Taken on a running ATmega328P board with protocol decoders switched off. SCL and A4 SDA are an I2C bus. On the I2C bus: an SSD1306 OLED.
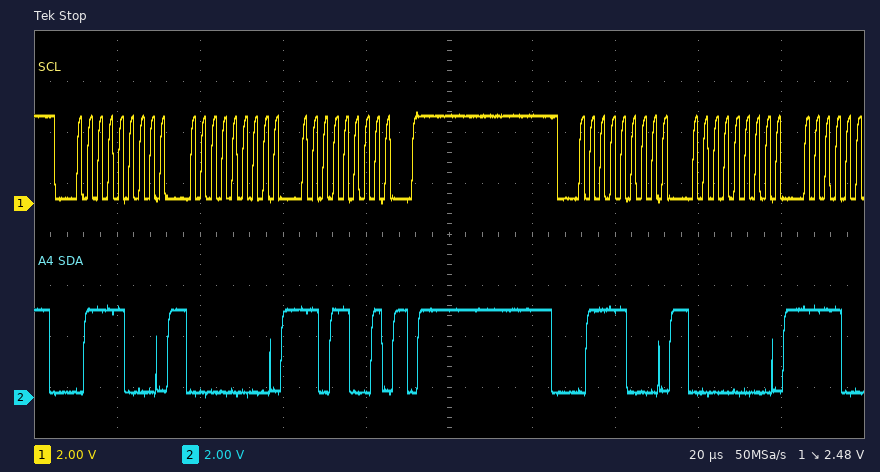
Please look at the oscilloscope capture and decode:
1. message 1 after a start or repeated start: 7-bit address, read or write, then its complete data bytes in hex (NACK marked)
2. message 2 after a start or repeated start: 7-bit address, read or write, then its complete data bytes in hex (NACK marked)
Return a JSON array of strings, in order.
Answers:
["0x3C write: 00 D9", "0x3C write: 00"]
